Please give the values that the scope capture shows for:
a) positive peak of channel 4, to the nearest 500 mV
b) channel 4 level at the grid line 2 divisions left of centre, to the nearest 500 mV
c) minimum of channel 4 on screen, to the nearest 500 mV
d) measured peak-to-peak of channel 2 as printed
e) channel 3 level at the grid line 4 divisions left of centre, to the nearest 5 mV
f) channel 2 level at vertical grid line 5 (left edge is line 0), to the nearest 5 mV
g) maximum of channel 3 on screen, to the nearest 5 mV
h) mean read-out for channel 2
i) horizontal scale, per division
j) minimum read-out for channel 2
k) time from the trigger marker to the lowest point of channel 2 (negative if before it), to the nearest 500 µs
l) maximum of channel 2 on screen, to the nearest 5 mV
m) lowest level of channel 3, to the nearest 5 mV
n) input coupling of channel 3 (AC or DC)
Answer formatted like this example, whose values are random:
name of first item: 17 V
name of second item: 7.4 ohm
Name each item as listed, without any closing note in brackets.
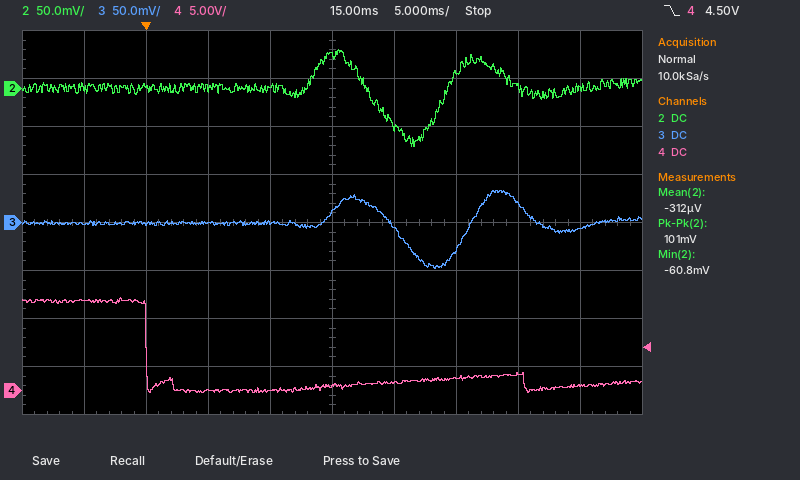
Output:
positive peak of channel 4, to the nearest 500 mV: 9.5 V
channel 4 level at the grid line 2 divisions left of centre, to the nearest 500 mV: 0.0 V
minimum of channel 4 on screen, to the nearest 500 mV: 0.0 V
measured peak-to-peak of channel 2 as printed: 101 mV
channel 3 level at the grid line 4 divisions left of centre, to the nearest 5 mV: 0 mV
channel 2 level at vertical grid line 5 (left edge is line 0), to the nearest 5 mV: 35 mV
maximum of channel 3 on screen, to the nearest 5 mV: 35 mV
mean read-out for channel 2: -312 µV
horizontal scale, per division: 5 ms
minimum read-out for channel 2: -60.8 mV
time from the trigger marker to the lowest point of channel 2 (negative if before it), to the nearest 500 µs: +21.5 ms
maximum of channel 2 on screen, to the nearest 5 mV: 40 mV
lowest level of channel 3, to the nearest 5 mV: -50 mV
input coupling of channel 3: DC
